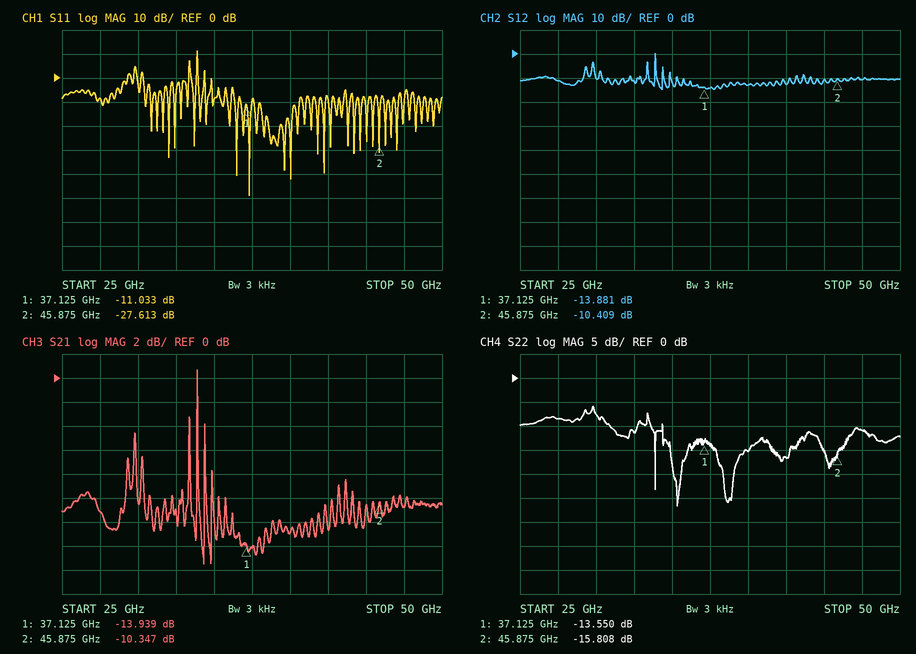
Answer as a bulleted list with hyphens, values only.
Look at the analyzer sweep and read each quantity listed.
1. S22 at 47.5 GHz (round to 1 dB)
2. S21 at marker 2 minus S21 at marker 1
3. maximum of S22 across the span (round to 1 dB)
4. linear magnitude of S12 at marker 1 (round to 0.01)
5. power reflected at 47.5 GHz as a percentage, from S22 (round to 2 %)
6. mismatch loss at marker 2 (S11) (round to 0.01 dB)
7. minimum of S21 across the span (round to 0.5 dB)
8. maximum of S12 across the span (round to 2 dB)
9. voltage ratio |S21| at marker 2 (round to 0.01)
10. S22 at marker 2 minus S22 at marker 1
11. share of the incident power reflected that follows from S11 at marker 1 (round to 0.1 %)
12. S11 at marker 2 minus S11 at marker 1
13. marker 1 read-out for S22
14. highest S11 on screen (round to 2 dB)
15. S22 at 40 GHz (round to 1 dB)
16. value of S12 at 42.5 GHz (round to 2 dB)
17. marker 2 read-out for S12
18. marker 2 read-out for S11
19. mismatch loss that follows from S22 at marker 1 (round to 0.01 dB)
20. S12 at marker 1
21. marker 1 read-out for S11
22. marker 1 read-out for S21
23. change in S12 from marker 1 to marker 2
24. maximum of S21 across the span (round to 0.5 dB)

- -11 dB
- 3.592 dB
- -6 dB
- 0.20
- 8 %
- 0.01 dB
- -15.5 dB
- 0 dB
- 0.30
- -2.258 dB
- 7.9 %
- -16.580 dB
- -13.550 dB
- 12 dB
- -15 dB
- -12 dB
- -10.409 dB
- -27.613 dB
- 0.20 dB
- -13.881 dB
- -11.033 dB
- -13.939 dB
- 3.472 dB
- 0.5 dB
